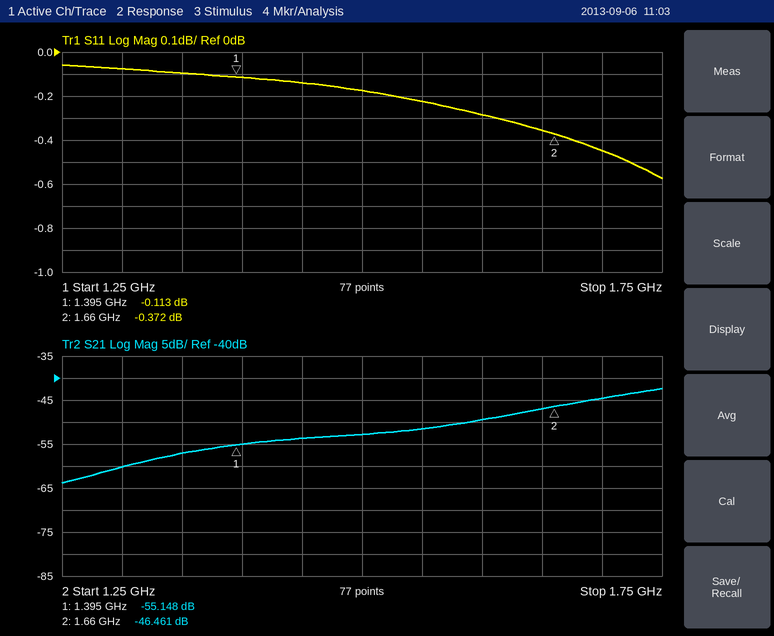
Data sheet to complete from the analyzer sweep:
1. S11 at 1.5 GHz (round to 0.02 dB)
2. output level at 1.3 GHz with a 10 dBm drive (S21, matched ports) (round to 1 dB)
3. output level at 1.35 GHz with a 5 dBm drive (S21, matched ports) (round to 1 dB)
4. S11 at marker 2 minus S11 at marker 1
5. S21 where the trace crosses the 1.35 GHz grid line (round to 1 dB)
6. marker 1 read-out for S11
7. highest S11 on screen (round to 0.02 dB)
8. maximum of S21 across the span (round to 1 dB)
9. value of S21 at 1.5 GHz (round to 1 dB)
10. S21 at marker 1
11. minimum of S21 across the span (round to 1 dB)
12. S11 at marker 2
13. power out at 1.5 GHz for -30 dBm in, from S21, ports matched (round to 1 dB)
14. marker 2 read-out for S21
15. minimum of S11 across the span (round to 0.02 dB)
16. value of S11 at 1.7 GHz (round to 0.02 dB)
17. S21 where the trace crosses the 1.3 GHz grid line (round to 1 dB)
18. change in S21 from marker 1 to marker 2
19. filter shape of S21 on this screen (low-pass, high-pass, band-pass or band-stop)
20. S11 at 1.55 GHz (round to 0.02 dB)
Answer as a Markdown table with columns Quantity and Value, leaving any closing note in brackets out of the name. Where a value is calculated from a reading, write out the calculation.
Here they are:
| Quantity | Value |
|---|---|
| S11 at 1.5 GHz | -0.18 dB |
| output level at 1.3 GHz with a 10 dBm drive (S21, matched ports) | 10 dBm + (-60 dB) = -50 dBm |
| output level at 1.35 GHz with a 5 dBm drive (S21, matched ports) | 5 dBm + (-57 dB) = -52 dBm |
| S11 at marker 2 minus S11 at marker 1 | -0.372 − (-0.113) = -0.259 dB |
| S21 where the trace crosses the 1.35 GHz grid line | -57 dB |
| marker 1 read-out for S11 | -0.113 dB |
| highest S11 on screen | -0.06 dB |
| maximum of S21 across the span | -42 dB |
| value of S21 at 1.5 GHz | -53 dB |
| S21 at marker 1 | -55.148 dB |
| minimum of S21 across the span | -64 dB |
| S11 at marker 2 | -0.372 dB |
| power out at 1.5 GHz for -30 dBm in, from S21, ports matched | -30 dBm + (-53 dB) = -83 dBm |
| marker 2 read-out for S21 | -46.461 dB |
| minimum of S11 across the span | -0.58 dB |
| value of S11 at 1.7 GHz | -0.44 dB |
| S21 where the trace crosses the 1.3 GHz grid line | -60 dB |
| change in S21 from marker 1 to marker 2 | -46.461 − (-55.148) = 8.687 dB |
| filter shape of S21 on this screen | high-pass |
| S11 at 1.55 GHz | -0.22 dB |
